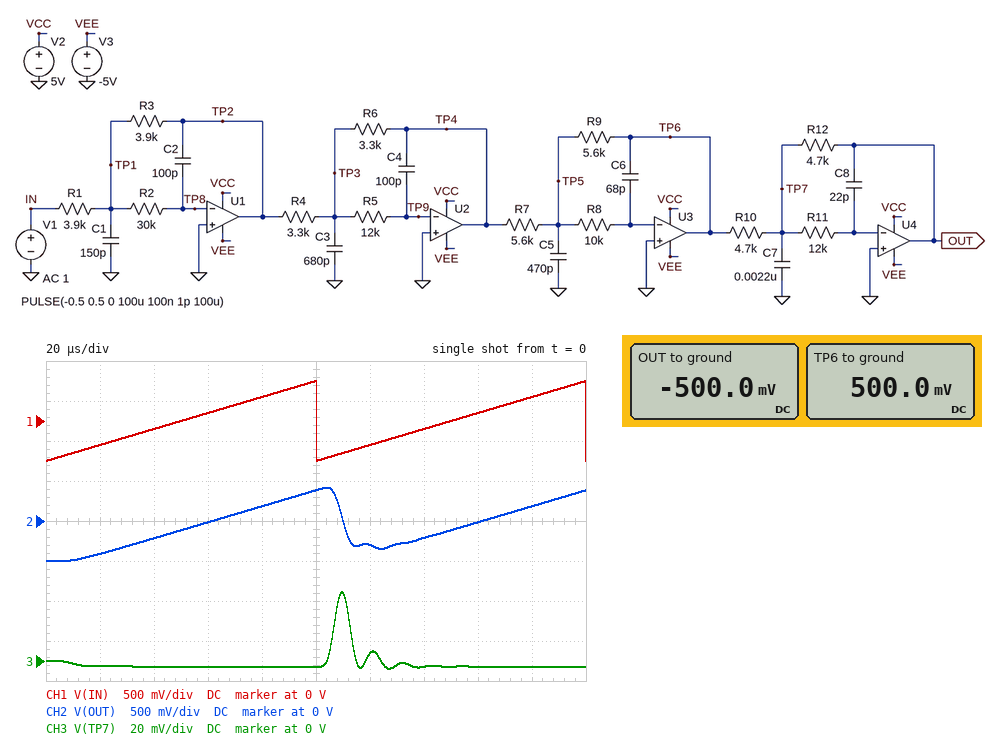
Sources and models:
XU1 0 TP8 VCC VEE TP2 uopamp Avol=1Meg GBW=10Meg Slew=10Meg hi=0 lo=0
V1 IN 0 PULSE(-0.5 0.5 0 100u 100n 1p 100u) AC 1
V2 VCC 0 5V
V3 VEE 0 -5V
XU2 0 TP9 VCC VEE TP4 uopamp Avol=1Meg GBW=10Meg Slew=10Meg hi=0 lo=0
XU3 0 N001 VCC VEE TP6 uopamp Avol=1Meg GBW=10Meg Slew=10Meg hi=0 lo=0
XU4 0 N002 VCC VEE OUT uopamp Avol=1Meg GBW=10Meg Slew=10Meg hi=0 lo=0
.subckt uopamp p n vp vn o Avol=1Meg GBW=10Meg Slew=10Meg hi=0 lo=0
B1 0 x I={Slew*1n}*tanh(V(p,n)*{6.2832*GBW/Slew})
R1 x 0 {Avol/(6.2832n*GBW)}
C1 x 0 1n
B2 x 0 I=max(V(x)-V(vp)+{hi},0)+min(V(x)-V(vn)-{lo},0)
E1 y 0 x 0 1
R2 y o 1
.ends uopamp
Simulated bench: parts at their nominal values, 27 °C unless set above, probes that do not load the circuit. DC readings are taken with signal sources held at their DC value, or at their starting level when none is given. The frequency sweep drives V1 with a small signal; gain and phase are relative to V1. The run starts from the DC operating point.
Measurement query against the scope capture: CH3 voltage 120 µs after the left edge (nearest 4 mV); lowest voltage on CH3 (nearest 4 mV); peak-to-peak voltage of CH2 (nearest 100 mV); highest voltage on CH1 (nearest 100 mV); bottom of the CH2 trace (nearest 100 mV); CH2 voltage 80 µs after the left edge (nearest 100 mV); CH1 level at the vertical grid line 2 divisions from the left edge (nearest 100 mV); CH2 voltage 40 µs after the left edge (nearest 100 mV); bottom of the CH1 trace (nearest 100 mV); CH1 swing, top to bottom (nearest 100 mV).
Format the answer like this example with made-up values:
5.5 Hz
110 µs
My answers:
4 mV
-4 mV
900 mV
500 mV
-500 mV
200 mV
-100 mV
-200 mV
-500 mV
1.0 V
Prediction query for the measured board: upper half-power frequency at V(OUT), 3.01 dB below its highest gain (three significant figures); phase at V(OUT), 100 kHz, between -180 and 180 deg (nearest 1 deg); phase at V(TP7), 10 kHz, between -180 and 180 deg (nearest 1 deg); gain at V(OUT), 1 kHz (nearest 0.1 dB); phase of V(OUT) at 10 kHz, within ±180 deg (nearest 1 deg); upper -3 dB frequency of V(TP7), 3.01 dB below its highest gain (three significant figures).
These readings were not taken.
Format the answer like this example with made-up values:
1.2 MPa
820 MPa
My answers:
29.3 kHz
-6 deg
-131 deg
0 dB
-41 deg
100 kHz
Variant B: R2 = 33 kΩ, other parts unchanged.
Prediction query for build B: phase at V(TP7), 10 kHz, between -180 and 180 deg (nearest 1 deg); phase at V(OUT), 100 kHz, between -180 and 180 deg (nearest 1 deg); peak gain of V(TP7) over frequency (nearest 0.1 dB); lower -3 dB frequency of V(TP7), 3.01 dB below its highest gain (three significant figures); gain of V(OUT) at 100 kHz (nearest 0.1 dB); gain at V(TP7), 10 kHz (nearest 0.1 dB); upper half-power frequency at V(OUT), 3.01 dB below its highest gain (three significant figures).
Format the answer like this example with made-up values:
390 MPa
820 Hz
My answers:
-133 deg
-7 deg
-23.7 dB
52.2 kHz
-11.5 dB
-35.7 dB
26.1 kHz
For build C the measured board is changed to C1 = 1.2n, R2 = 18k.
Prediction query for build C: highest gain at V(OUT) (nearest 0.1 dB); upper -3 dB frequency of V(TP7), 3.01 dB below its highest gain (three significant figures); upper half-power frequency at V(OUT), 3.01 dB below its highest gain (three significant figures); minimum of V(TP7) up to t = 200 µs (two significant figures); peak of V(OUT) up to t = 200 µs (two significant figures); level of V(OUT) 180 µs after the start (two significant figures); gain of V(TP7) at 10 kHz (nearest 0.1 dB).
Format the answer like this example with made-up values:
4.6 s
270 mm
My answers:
0.3 dB
97.0 kHz
75.6 kHz
-14 mV
450 mV
210 mV
-35.0 dB
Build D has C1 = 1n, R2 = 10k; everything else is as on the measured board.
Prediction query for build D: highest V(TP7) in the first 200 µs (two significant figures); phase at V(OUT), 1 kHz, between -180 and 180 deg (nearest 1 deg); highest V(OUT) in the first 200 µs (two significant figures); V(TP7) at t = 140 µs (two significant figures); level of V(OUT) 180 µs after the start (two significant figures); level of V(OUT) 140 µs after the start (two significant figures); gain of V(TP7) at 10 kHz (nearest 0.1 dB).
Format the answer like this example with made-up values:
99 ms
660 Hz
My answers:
64 mV
-3 deg
460 mV
-4.3 mV
220 mV
-170 mV
-35.0 dB
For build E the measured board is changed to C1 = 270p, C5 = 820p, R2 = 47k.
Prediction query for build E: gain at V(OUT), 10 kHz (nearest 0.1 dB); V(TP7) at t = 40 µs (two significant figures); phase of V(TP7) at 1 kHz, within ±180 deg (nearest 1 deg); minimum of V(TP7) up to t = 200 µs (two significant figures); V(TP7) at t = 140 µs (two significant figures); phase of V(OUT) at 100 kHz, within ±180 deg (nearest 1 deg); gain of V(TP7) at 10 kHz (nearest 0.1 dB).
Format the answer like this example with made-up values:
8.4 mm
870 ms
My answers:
-1.2 dB
-2.7 mV
-95 deg
-2.8 mV
-2.5 mV
-46 deg
-36.3 dB
